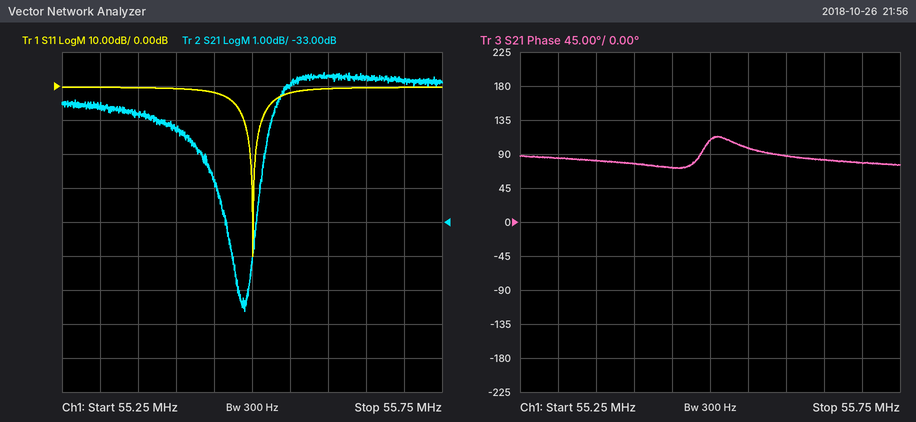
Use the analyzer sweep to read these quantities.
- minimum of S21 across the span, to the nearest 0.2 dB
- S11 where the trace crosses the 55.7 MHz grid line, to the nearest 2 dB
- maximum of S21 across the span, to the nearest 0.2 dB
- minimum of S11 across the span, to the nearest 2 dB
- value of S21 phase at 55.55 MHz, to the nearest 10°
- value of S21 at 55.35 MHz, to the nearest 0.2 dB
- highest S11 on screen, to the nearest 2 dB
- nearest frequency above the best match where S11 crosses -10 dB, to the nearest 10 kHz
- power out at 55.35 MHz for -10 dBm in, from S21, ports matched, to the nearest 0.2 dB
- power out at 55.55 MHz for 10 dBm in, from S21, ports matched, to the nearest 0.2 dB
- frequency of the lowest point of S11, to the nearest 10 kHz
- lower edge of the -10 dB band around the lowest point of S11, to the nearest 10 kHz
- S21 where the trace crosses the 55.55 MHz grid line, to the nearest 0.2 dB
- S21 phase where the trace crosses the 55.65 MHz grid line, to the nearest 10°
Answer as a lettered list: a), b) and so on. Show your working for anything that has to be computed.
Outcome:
a) -35.6 dB
b) 0 dB
c) -28.6 dB
d) -50 dB
e) 100°
f) -29.8 dB
g) 0 dB
h) 55.51 MHz
i) -10 dBm + (-29.8 dB) = -39.8 dBm
j) 10 dBm + (-29.0 dB) = -19.0 dBm
k) 55.50 MHz
l) 55.49 MHz
m) -29.0 dB
n) 80°
